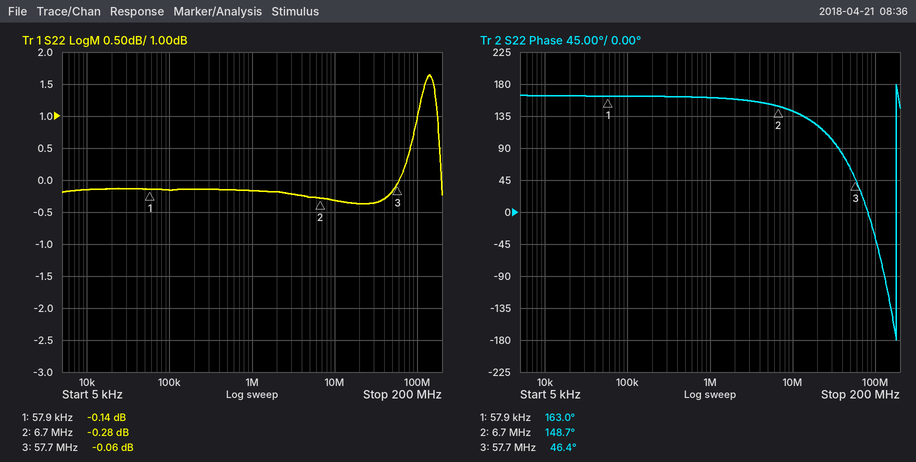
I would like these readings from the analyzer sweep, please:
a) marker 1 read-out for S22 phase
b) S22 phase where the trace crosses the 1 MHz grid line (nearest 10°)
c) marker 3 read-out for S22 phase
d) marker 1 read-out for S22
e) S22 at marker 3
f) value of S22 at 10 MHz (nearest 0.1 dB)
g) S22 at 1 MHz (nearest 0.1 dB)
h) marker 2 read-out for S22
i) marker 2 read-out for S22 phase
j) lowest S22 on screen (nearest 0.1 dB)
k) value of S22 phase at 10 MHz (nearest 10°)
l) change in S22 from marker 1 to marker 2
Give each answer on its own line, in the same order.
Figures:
163.0°
160°
46.4°
-0.14 dB
-0.06 dB
-0.3 dB
-0.2 dB
-0.28 dB
148.7°
-0.4 dB
140°
-0.14 dB
